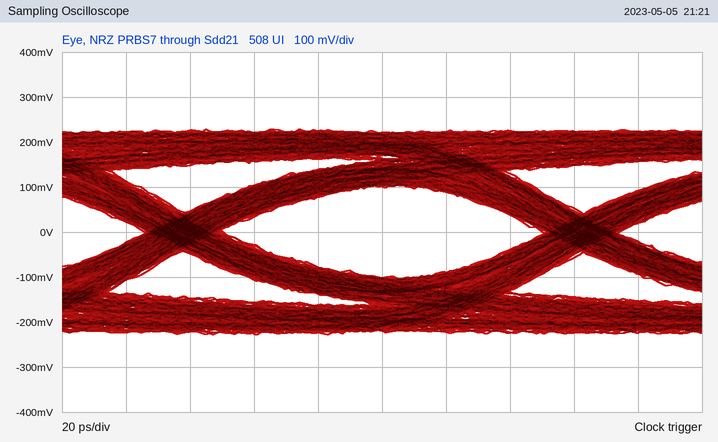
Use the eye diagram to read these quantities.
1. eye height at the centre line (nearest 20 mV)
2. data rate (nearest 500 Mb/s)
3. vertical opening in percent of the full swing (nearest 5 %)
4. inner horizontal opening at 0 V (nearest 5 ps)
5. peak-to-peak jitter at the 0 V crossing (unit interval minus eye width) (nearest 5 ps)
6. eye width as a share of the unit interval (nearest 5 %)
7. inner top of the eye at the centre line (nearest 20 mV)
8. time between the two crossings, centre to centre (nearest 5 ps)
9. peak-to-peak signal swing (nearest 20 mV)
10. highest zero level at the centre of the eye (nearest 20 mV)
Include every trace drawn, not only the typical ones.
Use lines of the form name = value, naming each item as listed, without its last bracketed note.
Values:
eye height at the centre line = 200 mV
data rate = 8.0 Gb/s
vertical opening in percent of the full swing = 45 %
inner horizontal opening at 0 V = 100 ps
peak-to-peak jitter at the 0 V crossing (unit interval minus eye width) = 25 ps
eye width as a share of the unit interval = 80 %
inner top of the eye at the centre line = 100 mV
time between the two crossings, centre to centre = 125 ps
peak-to-peak signal swing = 460 mV
highest zero level at the centre of the eye = -100 mV
